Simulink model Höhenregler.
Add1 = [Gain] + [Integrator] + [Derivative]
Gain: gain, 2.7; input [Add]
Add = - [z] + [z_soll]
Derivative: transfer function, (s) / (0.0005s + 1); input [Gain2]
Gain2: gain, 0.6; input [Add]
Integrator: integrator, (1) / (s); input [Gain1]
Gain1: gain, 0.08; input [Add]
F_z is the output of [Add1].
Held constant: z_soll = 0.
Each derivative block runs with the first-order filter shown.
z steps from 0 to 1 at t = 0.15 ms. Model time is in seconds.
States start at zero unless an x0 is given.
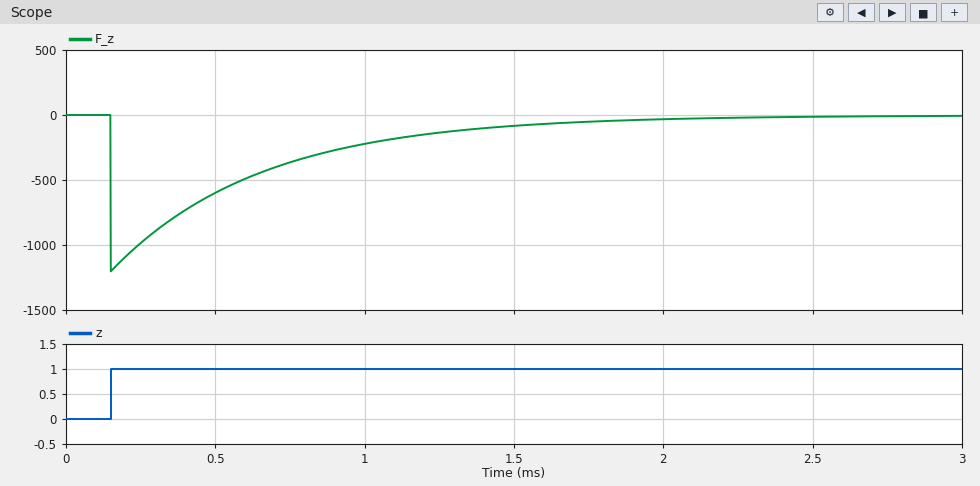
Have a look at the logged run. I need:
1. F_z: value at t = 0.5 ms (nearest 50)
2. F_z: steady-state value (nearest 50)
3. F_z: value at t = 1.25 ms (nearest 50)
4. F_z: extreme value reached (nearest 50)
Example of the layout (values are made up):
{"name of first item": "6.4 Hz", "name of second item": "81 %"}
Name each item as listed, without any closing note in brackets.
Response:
{"F_z: value at t = 0.5 ms": "-600", "F_z: steady-state value": "0", "F_z: value at t = 1.25 ms": "-150", "F_z: extreme value reached": "-1200"}
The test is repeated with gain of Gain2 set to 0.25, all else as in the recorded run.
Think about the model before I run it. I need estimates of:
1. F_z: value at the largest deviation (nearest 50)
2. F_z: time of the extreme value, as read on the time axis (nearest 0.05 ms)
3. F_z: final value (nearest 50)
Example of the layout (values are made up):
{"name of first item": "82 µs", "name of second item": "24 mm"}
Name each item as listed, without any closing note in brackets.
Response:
{"F_z: value at the largest deviation": "-500", "F_z: time of the extreme value, as read on the time axis": "0.15 ms", "F_z: final value": "0"}
